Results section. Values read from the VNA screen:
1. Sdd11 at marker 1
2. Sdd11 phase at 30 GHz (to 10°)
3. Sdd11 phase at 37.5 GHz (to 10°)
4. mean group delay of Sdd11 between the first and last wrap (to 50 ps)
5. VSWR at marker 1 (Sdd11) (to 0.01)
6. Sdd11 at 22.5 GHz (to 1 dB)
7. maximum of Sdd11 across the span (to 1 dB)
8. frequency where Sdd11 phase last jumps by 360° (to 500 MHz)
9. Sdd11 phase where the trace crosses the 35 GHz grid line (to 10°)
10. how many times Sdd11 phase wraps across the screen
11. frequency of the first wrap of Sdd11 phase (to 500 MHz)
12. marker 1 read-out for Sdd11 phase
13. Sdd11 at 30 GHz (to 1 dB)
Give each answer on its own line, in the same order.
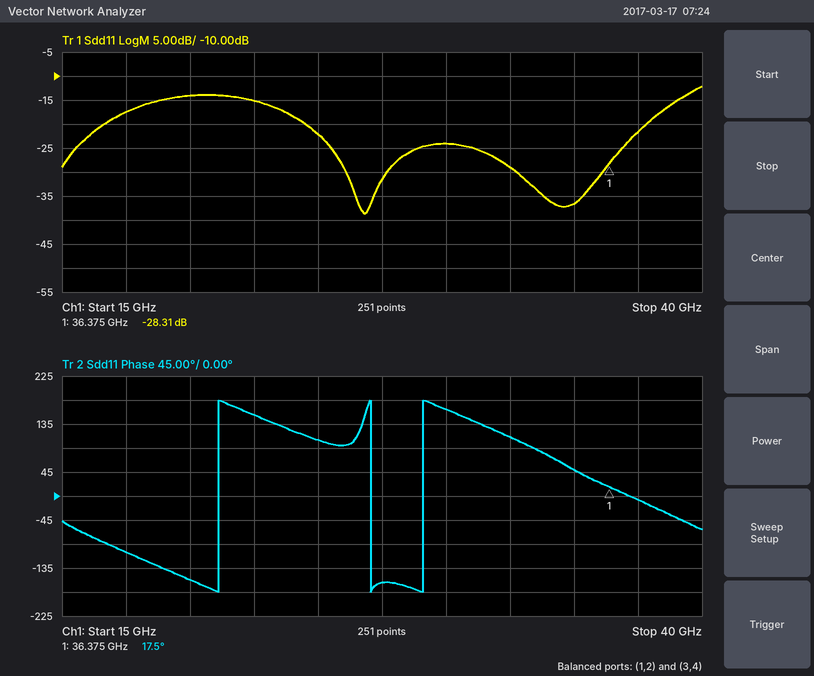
-28.31 dB
160°
-10°
250 ps
1.08
-15 dB
-12 dB
29.0 GHz
50°
3
21.0 GHz
17.5°
-24 dB
